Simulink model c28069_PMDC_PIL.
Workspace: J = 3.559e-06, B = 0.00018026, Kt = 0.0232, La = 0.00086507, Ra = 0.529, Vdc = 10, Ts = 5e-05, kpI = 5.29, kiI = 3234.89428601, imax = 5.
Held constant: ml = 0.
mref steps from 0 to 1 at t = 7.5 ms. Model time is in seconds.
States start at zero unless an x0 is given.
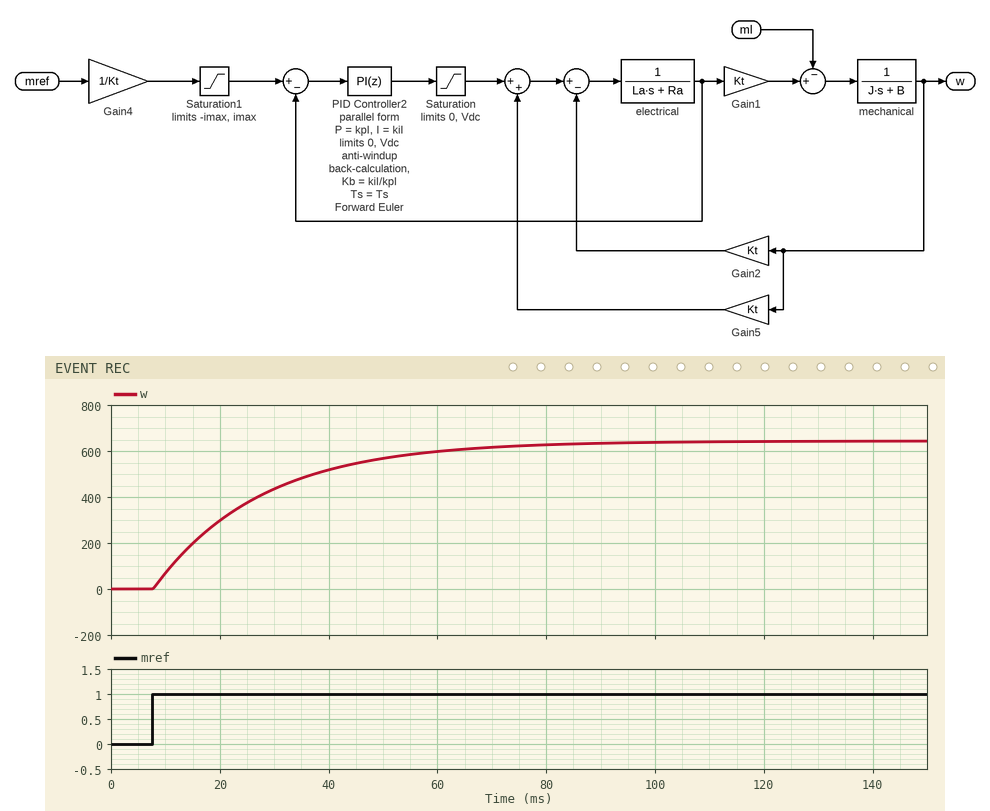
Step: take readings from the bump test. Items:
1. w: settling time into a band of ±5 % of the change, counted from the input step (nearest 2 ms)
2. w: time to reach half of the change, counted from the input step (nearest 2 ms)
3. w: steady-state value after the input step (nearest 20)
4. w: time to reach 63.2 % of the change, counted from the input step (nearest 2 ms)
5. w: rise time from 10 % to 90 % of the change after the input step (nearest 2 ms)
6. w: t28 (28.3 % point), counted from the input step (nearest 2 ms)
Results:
60 ms
14 ms
640
20 ms
44 ms
6 ms
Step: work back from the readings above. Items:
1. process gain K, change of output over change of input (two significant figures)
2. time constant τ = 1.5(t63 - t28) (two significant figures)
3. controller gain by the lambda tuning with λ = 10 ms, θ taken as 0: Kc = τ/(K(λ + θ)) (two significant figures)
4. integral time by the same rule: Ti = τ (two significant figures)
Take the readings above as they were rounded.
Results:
640
21 ms
0.0033
21 ms
